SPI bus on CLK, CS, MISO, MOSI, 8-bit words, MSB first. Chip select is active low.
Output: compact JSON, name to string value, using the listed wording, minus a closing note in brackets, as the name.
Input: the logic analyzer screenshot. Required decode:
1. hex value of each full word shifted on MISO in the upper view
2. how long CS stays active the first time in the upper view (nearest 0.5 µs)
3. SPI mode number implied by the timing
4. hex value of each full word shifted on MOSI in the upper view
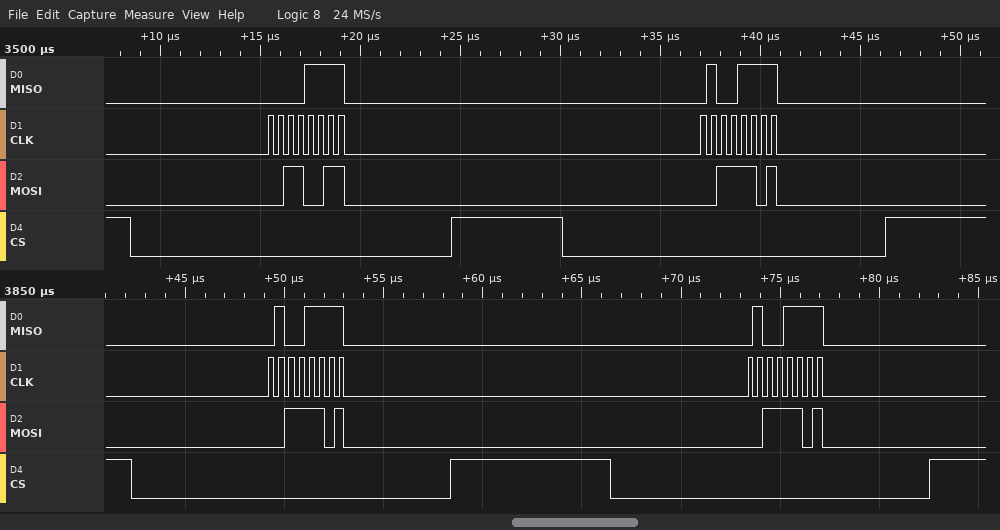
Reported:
{"hex value of each full word shifted on MISO in the upper view": "0F, 4F", "how long CS stays active the first time in the upper view": "16 µs", "SPI mode number implied by the timing": "0", "hex value of each full word shifted on MOSI in the upper view": "33, 3D"}
